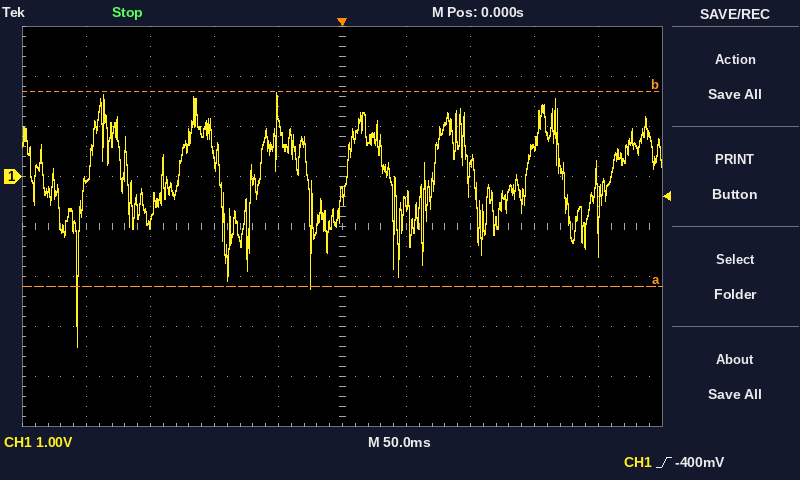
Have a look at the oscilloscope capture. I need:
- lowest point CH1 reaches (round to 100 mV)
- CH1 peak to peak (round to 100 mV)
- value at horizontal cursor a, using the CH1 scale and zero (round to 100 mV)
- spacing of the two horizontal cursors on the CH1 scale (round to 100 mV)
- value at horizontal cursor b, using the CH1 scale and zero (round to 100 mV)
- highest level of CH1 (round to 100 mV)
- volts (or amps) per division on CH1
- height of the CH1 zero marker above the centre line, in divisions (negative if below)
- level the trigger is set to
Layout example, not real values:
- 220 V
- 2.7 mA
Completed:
- -3.4 V
- 5.1 V
- -2.2 V
- 3.9 V
- 1.7 V
- 1.7 V
- 1 V
- +1.0 div
- -400 mV
